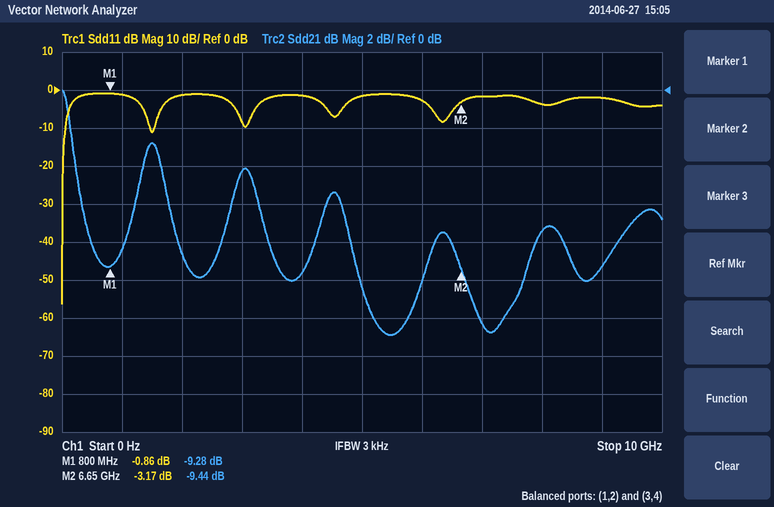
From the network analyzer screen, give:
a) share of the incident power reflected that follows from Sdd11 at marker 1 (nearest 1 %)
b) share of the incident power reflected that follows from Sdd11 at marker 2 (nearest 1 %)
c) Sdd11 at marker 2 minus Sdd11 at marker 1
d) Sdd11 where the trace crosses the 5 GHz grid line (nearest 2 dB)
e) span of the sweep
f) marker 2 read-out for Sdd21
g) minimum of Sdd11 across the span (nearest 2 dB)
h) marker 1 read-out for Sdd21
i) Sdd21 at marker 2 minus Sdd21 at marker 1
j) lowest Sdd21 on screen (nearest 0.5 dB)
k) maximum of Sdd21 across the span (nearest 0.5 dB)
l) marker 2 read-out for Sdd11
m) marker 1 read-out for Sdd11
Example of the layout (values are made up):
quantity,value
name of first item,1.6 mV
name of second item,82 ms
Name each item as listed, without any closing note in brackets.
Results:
quantity,value
share of the incident power reflected that follows from Sdd11 at marker 1,82 %
share of the incident power reflected that follows from Sdd11 at marker 2,48 %
Sdd11 at marker 2 minus Sdd11 at marker 1,-2.31 dB
Sdd11 where the trace crosses the 5 GHz grid line,-2 dB
span of the sweep,10 GHz
marker 2 read-out for Sdd21,-9.44 dB
minimum of Sdd11 across the span,-56 dB
marker 1 read-out for Sdd21,-9.28 dB
Sdd21 at marker 2 minus Sdd21 at marker 1,-0.16 dB
lowest Sdd21 on screen,-13.0 dB
maximum of Sdd21 across the span,0.0 dB
marker 2 read-out for Sdd11,-3.17 dB
marker 1 read-out for Sdd11,-0.86 dB
